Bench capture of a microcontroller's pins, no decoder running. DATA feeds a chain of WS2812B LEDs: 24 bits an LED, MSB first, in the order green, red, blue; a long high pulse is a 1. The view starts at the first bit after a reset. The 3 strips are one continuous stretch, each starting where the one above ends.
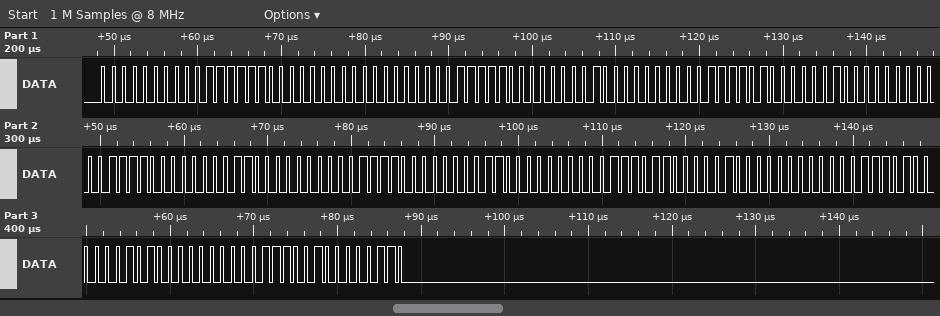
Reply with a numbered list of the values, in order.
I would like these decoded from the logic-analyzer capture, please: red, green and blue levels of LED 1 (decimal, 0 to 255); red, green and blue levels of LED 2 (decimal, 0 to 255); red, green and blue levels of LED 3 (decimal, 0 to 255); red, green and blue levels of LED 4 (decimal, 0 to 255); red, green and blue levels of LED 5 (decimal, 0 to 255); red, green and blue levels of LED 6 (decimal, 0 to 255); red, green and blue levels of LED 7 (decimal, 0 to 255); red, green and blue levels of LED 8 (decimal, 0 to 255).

1. 63, 0, 0
2. 62, 0, 1
3. 61, 0, 2
4. 60, 0, 3
5. 60, 0, 3
6. 59, 0, 4
7. 58, 0, 5
8. 57, 0, 6
